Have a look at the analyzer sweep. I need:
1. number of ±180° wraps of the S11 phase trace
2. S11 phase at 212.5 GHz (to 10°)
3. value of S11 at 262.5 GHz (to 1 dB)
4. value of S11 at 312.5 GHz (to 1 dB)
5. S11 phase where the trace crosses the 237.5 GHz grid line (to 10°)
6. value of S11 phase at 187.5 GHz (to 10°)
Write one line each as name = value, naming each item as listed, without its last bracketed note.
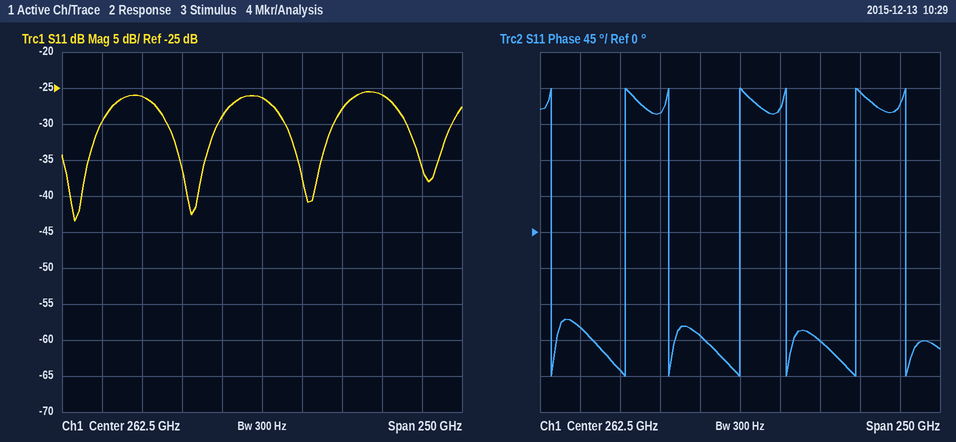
number of ±180° wraps of the S11 phase trace = 7
S11 phase at 212.5 GHz = 150°
value of S11 at 262.5 GHz = -26 dB
value of S11 at 312.5 GHz = -28 dB
S11 phase where the trace crosses the 237.5 GHz grid line = -130°
value of S11 phase at 187.5 GHz = -170°
